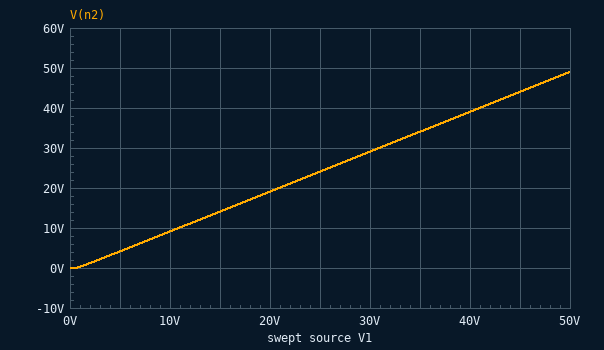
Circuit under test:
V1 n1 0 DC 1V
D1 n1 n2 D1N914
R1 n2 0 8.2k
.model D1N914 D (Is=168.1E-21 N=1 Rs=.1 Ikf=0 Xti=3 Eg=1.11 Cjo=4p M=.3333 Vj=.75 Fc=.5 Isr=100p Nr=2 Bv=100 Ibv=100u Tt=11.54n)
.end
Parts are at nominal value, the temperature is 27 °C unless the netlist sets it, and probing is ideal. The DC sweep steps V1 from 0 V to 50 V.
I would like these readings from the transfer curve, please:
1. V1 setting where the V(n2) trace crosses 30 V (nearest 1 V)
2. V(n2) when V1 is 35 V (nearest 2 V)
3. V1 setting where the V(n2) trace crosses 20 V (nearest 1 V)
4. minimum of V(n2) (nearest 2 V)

31 V
34 V
21 V
0 V
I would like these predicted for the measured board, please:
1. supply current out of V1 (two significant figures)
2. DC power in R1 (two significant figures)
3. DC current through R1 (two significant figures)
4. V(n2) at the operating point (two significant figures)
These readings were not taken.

36 µA
11 µW
36 µA
300 mV
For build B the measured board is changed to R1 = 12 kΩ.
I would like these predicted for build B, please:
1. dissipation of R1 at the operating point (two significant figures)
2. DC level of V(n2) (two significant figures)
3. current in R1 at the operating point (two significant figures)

8.4 µW
320 mV
26 µA
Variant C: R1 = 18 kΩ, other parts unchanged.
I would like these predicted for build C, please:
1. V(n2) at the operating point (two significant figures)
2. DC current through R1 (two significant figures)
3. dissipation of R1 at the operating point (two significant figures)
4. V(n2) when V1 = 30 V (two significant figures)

340 mV
19 µA
6.3 µW
29 V
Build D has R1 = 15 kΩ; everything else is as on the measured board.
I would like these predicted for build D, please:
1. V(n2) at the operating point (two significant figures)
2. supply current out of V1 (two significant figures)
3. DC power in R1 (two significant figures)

330 mV
22 µA
7.2 µW
